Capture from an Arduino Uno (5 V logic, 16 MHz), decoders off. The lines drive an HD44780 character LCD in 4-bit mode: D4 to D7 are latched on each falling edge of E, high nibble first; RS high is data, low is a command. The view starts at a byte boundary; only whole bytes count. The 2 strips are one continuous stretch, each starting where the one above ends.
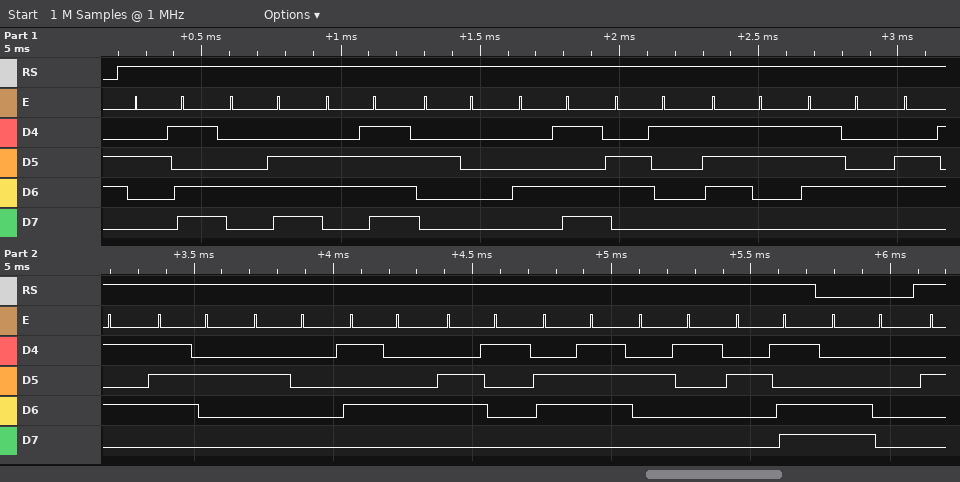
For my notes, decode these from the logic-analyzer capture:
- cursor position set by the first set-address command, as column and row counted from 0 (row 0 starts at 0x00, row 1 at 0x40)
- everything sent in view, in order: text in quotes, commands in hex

column 0, row 1
"-No Master Tag!-" 0xC0
